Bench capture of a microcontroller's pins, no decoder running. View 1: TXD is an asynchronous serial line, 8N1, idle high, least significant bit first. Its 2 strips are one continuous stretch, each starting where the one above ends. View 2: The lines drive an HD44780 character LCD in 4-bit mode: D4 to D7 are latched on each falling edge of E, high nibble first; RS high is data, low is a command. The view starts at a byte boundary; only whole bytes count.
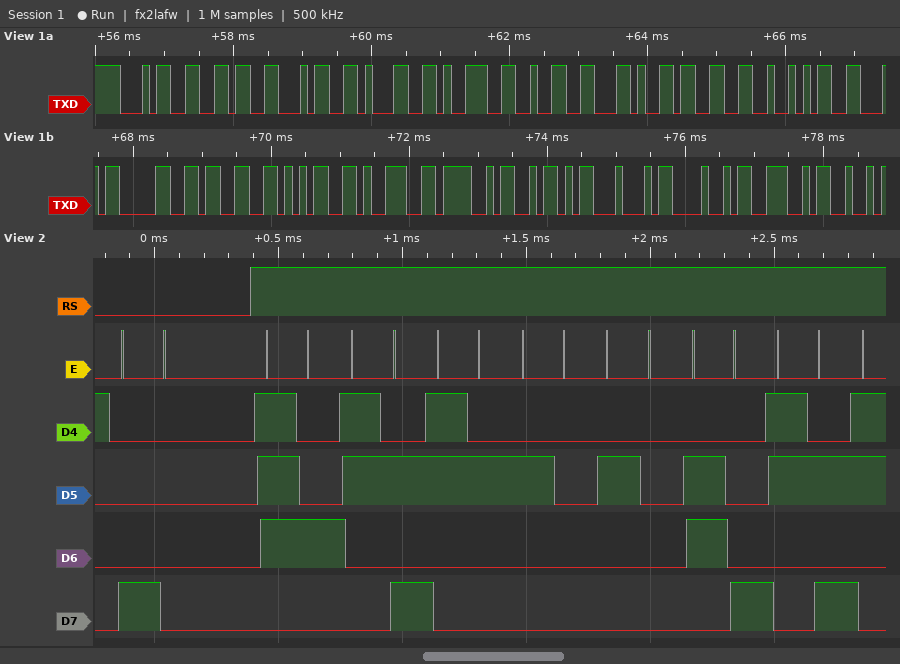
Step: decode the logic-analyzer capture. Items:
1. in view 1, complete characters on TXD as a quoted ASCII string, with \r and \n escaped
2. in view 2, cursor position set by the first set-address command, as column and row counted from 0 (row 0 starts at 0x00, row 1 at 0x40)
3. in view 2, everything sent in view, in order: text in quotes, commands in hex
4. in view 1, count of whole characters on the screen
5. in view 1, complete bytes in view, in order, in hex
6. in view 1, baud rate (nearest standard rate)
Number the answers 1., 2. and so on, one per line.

1. "464192,3RF0359OZDHN"
2. column 0, row 0
3. 0x80 "t:2  h:"
4. 19
5. 34 36 34 31 39 32 2C 33 52 46 30 33 35 39 4F 5A 44 48 4E
6. 9600 baud
